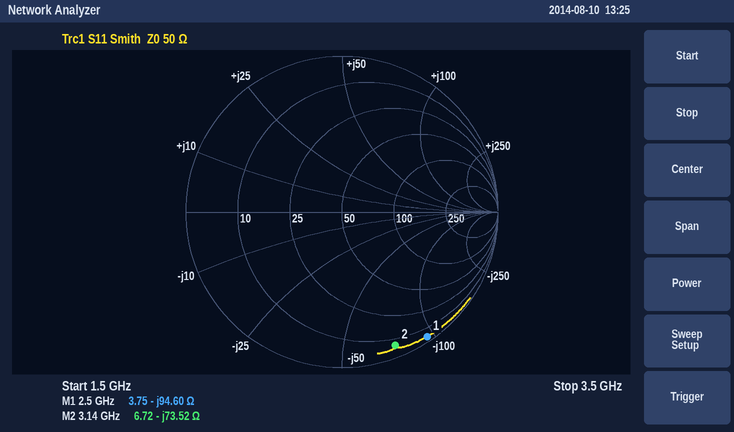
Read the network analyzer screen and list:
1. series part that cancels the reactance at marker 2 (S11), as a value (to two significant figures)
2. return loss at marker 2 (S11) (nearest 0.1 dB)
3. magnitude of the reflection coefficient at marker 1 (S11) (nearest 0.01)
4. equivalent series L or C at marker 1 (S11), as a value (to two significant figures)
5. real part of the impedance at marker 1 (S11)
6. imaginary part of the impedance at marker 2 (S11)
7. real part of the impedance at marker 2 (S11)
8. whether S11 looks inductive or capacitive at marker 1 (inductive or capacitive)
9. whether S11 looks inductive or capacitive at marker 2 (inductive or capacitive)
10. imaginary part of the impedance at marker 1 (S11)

3.7 nH
0.7 dB
0.97
670 fF
3.75 Ω
-73.52 Ω
6.72 Ω
capacitive
capacitive
-94.60 Ω
